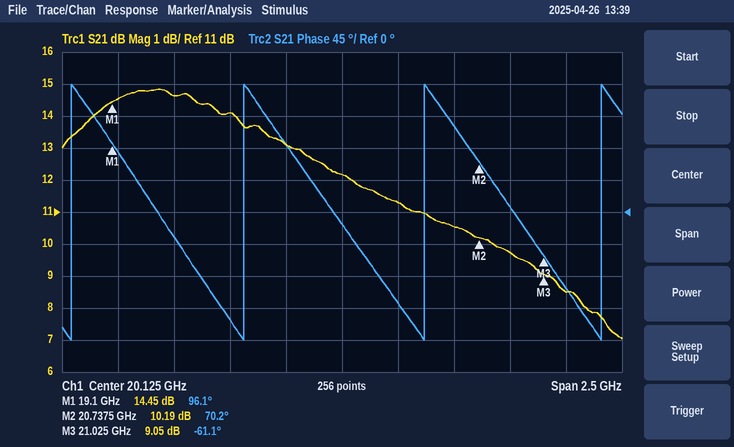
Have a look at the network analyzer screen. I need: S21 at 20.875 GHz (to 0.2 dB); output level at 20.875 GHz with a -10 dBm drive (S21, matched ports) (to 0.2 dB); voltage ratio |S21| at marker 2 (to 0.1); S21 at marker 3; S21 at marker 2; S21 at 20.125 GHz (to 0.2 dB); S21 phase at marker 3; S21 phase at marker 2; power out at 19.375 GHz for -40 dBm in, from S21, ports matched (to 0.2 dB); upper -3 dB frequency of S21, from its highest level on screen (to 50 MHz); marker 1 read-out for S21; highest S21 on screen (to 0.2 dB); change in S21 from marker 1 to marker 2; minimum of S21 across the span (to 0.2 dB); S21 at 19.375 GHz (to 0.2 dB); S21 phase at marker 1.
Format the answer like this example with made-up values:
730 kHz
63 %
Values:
9.8 dB
-0.2 dBm
3.2
9.05 dB
10.19 dB
12.2 dB
-61.1°
70.2°
-25.4 dBm
20.20 GHz
14.45 dB
14.8 dB
-4.26 dB
7.0 dB
14.6 dB
96.1°
